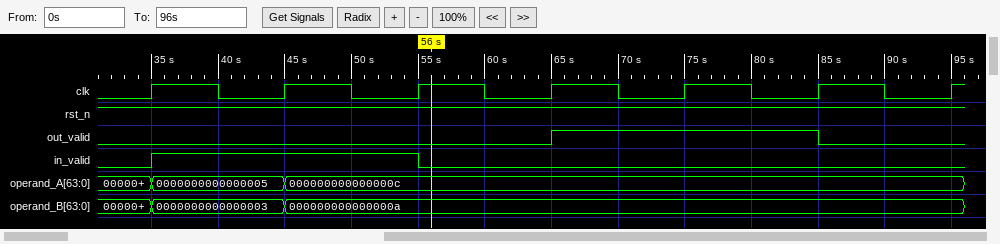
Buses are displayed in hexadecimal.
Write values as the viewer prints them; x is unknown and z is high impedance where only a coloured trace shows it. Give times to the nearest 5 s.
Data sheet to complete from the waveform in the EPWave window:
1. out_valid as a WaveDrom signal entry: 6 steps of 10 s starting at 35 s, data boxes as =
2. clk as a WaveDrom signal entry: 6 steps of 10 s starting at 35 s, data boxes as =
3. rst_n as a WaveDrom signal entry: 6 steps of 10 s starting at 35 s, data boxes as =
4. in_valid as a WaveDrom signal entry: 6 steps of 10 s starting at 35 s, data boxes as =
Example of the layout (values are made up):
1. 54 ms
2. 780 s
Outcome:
1. {name: 'out_valid', wave: '0..1.0'}
2. {name: 'clk', wave: 'p.....'}
3. {name: 'rst_n', wave: '1.....'}
4. {name: 'in_valid', wave: '1.0...'}
